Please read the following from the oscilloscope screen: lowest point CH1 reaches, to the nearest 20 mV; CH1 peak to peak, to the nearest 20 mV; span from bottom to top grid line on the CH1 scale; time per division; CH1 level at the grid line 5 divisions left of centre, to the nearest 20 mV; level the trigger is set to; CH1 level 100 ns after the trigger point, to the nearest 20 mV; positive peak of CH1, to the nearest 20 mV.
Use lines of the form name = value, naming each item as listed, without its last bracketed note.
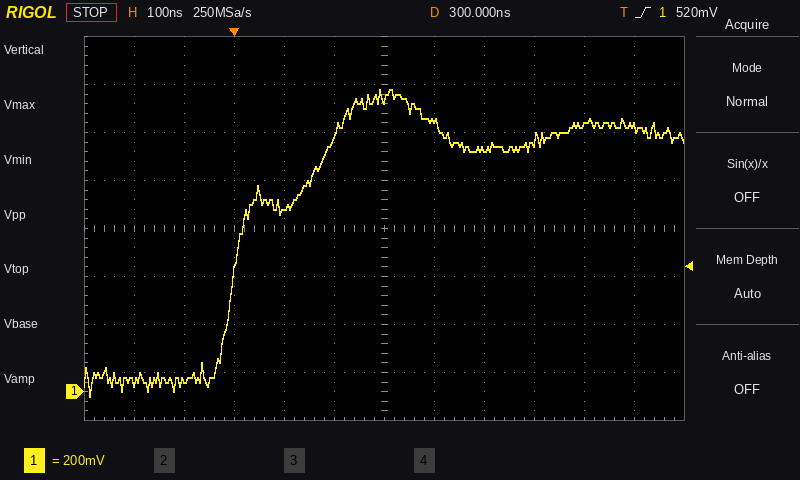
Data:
lowest point CH1 reaches, to the nearest 20 mV = -20 mV
CH1 peak to peak, to the nearest 20 mV = 1.28 V
span from bottom to top grid line on the CH1 scale = 1.6 V
time per division = 100 ns
CH1 level at the grid line 5 divisions left of centre, to the nearest 20 mV = 40 mV
level the trigger is set to = 520 mV
CH1 level 100 ns after the trigger point, to the nearest 20 mV = 760 mV
positive peak of CH1, to the nearest 20 mV = 1.26 V
